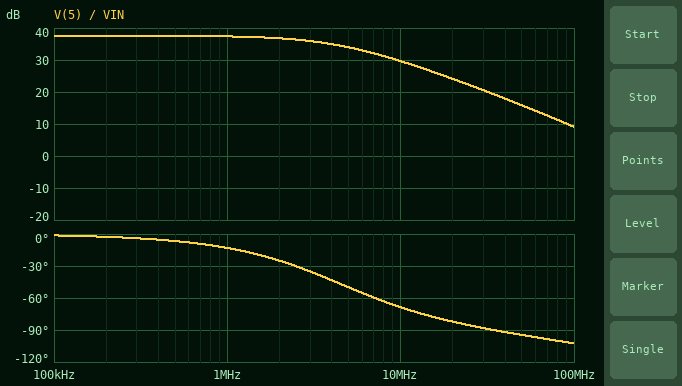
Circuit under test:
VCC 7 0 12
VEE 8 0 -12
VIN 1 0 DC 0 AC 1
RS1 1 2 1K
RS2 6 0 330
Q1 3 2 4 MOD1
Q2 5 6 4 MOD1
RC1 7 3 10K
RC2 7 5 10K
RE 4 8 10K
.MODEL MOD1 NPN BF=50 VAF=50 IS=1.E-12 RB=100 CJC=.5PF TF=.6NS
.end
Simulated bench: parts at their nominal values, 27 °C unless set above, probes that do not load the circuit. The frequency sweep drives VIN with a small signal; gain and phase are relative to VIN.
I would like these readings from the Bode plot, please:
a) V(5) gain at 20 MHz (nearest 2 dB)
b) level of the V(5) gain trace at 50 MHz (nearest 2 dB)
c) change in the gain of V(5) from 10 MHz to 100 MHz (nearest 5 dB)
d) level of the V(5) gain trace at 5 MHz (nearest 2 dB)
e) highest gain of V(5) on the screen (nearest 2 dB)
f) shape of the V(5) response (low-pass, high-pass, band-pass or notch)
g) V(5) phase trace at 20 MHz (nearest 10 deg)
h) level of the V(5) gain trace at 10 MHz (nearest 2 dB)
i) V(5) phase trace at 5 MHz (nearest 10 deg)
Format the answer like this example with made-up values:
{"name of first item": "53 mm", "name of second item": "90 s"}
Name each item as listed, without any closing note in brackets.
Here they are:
{"V(5) gain at 20 MHz": "24 dB", "level of the V(5) gain trace at 50 MHz": "16 dB", "change in the gain of V(5) from 10 MHz to 100 MHz": "-20 dB", "level of the V(5) gain trace at 5 MHz": "34 dB", "highest gain of V(5) on the screen": "38 dB", "shape of the V(5) response": "low-pass", "V(5) phase trace at 20 MHz": "-80 deg", "level of the V(5) gain trace at 10 MHz": "30 dB", "V(5) phase trace at 5 MHz": "-50 deg"}
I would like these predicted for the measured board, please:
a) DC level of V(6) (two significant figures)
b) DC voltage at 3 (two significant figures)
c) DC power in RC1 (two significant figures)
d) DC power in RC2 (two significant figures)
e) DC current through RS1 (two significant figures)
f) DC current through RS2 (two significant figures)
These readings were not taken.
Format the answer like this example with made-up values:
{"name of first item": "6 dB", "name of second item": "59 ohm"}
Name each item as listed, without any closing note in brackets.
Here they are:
{"DC level of V(6)": "-3.6 mV", "DC voltage at 3": "6.9 V", "DC power in RC1": "2.6 mW", "DC power in RC2": "3.8 mW", "DC current through RS1": "9.0 µA", "DC current through RS2": "11 µA"}
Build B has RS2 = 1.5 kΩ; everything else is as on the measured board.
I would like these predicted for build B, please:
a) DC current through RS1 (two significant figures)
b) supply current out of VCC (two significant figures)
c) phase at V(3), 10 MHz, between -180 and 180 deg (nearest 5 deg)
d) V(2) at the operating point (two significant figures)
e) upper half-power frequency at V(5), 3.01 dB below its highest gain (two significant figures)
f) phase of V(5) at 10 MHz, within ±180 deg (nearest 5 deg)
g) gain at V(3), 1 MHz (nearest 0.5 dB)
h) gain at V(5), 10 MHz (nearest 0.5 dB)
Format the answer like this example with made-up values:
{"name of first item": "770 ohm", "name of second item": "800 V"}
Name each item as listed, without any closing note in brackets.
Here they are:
{"DC current through RS1": "11 µA", "supply current out of VCC": "1.1 mA", "phase at V(3), 10 MHz, between -180 and 180 deg": "105 deg", "V(2) at the operating point": "-11 mV", "upper half-power frequency at V(5), 3.01 dB below its highest gain": "2.9 MHz", "phase of V(5) at 10 MHz, within ±180 deg": "-75 deg", "gain at V(3), 1 MHz": "36.0 dB", "gain at V(5), 10 MHz": "25.0 dB"}
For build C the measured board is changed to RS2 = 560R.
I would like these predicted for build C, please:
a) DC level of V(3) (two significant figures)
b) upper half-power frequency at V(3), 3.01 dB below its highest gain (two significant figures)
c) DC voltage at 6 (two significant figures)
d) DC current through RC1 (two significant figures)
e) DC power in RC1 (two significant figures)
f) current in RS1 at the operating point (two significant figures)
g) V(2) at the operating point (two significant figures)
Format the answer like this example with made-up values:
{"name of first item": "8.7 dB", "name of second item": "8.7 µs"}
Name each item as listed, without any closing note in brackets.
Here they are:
{"DC level of V(3)": "6.7 V", "upper half-power frequency at V(3), 3.01 dB below its highest gain": "3.9 MHz", "DC voltage at 6": "-6.0 mV", "DC current through RC1": "530 µA", "DC power in RC1": "2.8 mW", "current in RS1 at the operating point": "9.4 µA", "V(2) at the operating point": "-9.4 mV"}
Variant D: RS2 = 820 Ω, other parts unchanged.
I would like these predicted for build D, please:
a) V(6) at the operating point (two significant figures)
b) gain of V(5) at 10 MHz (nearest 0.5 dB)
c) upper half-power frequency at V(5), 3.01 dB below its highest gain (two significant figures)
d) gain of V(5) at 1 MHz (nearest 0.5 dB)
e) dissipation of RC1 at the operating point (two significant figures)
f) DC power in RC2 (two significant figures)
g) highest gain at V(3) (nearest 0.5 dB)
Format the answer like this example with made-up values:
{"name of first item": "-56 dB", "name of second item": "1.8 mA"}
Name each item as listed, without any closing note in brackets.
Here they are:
{"V(6) at the operating point": "-8.4 mV", "gain of V(5) at 10 MHz": "27.5 dB", "upper half-power frequency at V(5), 3.01 dB below its highest gain": "3.6 MHz", "gain of V(5) at 1 MHz": "36.5 dB", "dissipation of RC1 at the operating point": "3.0 mW", "DC power in RC2": "3.3 mW", "highest gain at V(3)": "37.0 dB"}
